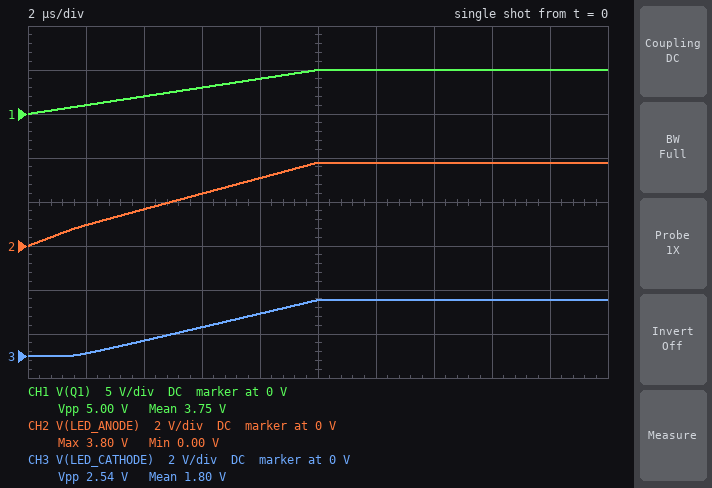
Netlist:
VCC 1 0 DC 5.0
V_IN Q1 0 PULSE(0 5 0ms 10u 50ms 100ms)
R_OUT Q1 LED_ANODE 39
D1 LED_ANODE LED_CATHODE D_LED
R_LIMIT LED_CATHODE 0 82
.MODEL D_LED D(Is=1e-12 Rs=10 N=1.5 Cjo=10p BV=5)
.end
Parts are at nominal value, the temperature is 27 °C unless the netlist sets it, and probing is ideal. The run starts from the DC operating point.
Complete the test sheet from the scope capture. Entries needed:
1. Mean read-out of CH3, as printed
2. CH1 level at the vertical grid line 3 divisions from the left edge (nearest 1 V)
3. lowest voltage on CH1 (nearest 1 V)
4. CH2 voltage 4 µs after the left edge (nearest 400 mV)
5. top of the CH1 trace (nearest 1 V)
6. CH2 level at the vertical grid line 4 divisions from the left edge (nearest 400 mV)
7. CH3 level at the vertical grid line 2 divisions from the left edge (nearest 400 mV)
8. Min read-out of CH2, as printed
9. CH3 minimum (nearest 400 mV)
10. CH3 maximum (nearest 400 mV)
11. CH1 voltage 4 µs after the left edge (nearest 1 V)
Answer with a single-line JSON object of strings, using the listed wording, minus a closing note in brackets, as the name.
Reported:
{"Mean read-out of CH3, as printed": "1.80 V", "CH1 level at the vertical grid line 3 divisions from the left edge": "3 V", "lowest voltage on CH1": "0 V", "CH2 voltage 4 µs after the left edge": "1.6 V", "top of the CH1 trace": "5 V", "CH2 level at the vertical grid line 4 divisions from the left edge": "3.2 V", "CH3 level at the vertical grid line 2 divisions from the left edge": "800 mV", "Min read-out of CH2, as printed": "0.00 V", "CH3 minimum": "0 V", "CH3 maximum": "2.4 V", "CH1 voltage 4 µs after the left edge": "2 V"}
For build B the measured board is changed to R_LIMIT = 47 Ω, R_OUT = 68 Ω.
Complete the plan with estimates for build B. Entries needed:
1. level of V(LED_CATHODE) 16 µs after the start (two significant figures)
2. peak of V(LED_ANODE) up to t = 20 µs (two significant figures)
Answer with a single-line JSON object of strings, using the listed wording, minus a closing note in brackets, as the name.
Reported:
{"level of V(LED_CATHODE) 16 µs after the start": "1.5 V", "peak of V(LED_ANODE) up to t = 20 µs": "2.8 V"}
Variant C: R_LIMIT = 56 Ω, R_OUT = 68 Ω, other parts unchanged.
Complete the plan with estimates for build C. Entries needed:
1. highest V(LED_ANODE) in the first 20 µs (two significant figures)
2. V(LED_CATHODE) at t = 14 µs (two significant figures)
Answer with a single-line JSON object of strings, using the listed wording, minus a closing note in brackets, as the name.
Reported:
{"highest V(LED_ANODE) in the first 20 µs": "2.9 V", "V(LED_CATHODE) at t = 14 µs": "1.7 V"}
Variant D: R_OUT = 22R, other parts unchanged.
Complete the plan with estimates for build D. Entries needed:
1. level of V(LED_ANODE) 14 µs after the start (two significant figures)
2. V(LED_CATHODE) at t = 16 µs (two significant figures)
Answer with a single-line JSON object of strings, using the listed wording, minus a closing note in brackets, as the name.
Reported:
{"level of V(LED_ANODE) 14 µs after the start": "4.2 V", "V(LED_CATHODE) at t = 16 µs": "2.9 V"}
